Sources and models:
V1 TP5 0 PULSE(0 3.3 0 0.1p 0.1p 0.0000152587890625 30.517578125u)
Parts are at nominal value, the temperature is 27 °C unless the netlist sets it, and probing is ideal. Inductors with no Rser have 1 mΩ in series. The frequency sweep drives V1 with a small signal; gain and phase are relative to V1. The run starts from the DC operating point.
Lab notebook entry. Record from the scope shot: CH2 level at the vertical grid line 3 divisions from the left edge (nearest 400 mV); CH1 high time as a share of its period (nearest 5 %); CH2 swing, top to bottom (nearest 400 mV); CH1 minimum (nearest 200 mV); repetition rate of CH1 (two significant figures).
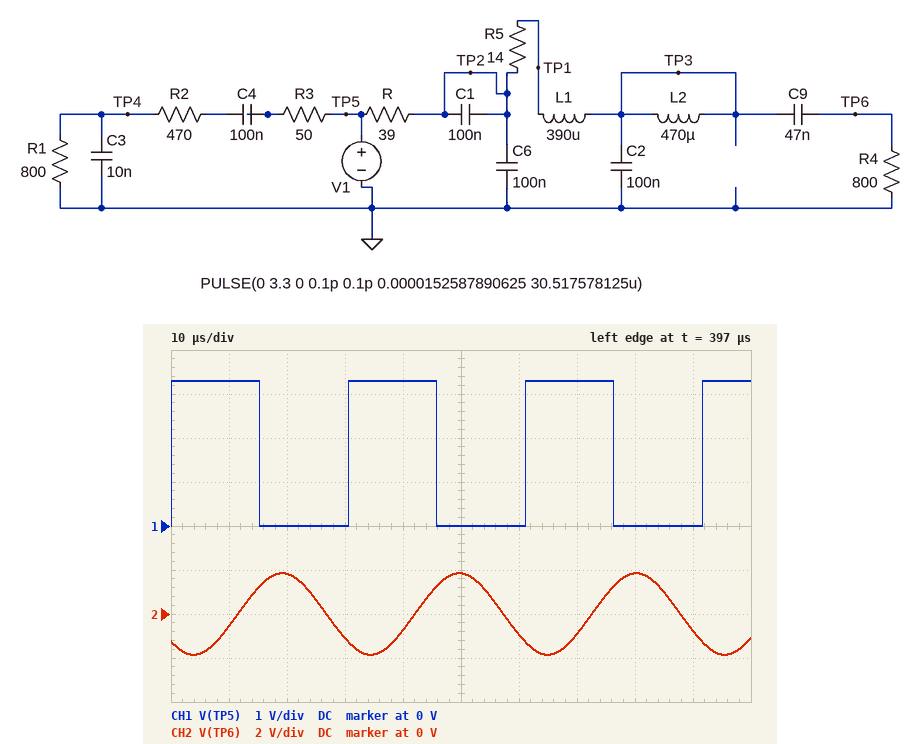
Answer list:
-1.2 V
50 %
3.6 V
0 V
33 kHz
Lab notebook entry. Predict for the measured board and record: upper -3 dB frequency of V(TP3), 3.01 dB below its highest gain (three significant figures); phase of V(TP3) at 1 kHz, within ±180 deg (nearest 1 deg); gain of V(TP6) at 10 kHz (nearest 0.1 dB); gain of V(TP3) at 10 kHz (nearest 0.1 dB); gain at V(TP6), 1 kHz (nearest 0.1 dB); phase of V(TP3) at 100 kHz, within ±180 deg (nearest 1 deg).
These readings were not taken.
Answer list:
35.5 kHz
-4 deg
-1.1 dB
-0.4 dB
-12.8 dB
119 deg
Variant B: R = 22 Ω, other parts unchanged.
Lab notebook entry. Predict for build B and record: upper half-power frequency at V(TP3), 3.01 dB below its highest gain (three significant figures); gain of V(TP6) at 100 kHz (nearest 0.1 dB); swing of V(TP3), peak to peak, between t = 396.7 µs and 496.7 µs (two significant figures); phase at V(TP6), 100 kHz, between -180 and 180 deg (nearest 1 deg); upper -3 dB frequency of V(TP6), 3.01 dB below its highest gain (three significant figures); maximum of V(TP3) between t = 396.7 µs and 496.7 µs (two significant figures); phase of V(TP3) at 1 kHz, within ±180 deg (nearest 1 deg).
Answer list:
32.3 kHz
-27.5 dB
4.4 V
135 deg
32.4 kHz
3.8 V
-3 deg
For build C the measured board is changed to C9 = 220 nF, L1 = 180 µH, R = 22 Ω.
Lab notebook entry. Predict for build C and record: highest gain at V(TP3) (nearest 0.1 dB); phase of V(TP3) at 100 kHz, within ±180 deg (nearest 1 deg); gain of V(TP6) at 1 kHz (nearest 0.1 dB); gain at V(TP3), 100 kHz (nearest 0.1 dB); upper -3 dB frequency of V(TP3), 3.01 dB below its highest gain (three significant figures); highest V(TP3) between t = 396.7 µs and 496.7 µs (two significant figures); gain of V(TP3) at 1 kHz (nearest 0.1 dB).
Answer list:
0.8 dB
141 deg
-2.8 dB
-19.6 dB
50.2 kHz
3.9 V
-0.2 dB
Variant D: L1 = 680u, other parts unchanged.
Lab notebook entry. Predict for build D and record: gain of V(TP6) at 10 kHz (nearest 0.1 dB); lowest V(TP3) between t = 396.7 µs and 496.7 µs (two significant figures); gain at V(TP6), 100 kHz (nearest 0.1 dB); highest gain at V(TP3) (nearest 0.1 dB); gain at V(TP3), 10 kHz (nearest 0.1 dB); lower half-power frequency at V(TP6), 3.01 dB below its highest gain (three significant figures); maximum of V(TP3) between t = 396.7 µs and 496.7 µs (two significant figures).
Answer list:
-0.1 dB
710 mV
-36.4 dB
2.4 dB
0.6 dB
8.07 kHz
2.6 V
